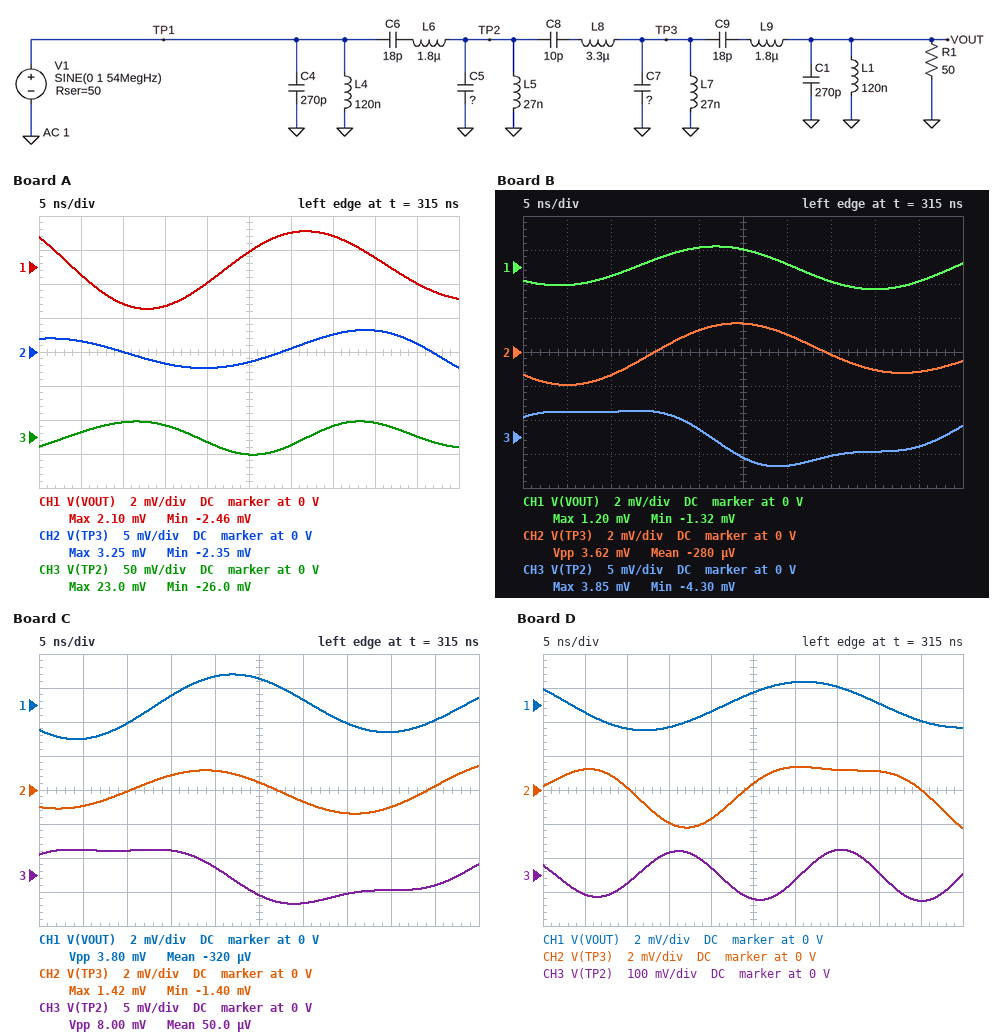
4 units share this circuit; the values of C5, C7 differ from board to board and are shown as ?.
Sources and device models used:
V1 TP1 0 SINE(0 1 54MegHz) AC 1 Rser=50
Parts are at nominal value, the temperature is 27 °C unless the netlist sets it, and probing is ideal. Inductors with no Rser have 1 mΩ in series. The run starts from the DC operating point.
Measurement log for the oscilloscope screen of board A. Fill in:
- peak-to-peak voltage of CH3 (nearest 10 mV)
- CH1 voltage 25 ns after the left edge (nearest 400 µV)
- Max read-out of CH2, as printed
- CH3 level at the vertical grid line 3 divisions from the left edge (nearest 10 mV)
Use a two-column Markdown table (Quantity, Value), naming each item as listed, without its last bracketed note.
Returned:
| Quantity | Value |
|---|---|
| peak-to-peak voltage of CH3 | 50 mV |
| CH1 voltage 25 ns after the left edge | 800 µV |
| Max read-out of CH2, as printed | 3.25 mV |
| CH3 level at the vertical grid line 3 divisions from the left edge | 20 mV |
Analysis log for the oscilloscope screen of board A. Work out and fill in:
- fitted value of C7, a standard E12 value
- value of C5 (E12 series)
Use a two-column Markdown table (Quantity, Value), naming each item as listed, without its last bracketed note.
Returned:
| Quantity | Value |
|---|---|
| fitted value of C7, a standard E12 value | 680 pF |
| value of C5 | 820 pF |
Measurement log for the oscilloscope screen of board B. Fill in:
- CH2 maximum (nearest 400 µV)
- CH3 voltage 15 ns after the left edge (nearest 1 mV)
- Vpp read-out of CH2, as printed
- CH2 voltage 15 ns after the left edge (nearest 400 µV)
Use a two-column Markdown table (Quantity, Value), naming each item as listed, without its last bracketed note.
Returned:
| Quantity | Value |
|---|---|
| CH2 maximum | 1.6 mV |
| CH3 voltage 15 ns after the left edge | 4 mV |
| Vpp read-out of CH2, as printed | 3.62 mV |
| CH2 voltage 15 ns after the left edge | 0 V |
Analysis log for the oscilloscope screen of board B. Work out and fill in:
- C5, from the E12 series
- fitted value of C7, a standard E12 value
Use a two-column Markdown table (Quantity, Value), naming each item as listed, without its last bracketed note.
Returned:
| Quantity | Value |
|---|---|
| C5, from the E12 series | 2.2 nF |
| fitted value of C7, a standard E12 value | 1.8 nF |
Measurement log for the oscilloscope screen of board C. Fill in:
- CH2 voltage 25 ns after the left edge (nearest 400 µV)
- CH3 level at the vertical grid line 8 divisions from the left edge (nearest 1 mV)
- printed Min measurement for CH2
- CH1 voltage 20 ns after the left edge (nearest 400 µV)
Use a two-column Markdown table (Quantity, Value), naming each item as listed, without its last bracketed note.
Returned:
| Quantity | Value |
|---|---|
| CH2 voltage 25 ns after the left edge | 400 µV |
| CH3 level at the vertical grid line 8 divisions from the left edge | -2 mV |
| printed Min measurement for CH2 | -1.40 mV |
| CH1 voltage 20 ns after the left edge | 1.6 mV |
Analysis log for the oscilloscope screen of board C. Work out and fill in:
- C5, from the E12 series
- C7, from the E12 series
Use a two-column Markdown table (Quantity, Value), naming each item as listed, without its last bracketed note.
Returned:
| Quantity | Value |
|---|---|
| C5, from the E12 series | 2.2 nF |
| C7, from the E12 series | 1.5 nF |
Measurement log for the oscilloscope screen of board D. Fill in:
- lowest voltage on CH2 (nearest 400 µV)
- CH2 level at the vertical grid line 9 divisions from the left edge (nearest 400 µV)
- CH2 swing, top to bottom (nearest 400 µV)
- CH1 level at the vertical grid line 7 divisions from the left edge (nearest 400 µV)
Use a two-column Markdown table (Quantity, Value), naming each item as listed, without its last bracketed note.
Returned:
| Quantity | Value |
|---|---|
| lowest voltage on CH2 | -2.4 mV |
| CH2 level at the vertical grid line 9 divisions from the left edge | 0 V |
| CH2 swing, top to bottom | 3.6 mV |
| CH1 level at the vertical grid line 7 divisions from the left edge | 1.2 mV |
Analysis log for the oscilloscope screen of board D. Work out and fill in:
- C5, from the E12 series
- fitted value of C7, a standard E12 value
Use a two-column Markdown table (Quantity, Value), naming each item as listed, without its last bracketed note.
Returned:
| Quantity | Value |
|---|---|
| C5, from the E12 series | 390 pF |
| fitted value of C7, a standard E12 value | 680 pF |
